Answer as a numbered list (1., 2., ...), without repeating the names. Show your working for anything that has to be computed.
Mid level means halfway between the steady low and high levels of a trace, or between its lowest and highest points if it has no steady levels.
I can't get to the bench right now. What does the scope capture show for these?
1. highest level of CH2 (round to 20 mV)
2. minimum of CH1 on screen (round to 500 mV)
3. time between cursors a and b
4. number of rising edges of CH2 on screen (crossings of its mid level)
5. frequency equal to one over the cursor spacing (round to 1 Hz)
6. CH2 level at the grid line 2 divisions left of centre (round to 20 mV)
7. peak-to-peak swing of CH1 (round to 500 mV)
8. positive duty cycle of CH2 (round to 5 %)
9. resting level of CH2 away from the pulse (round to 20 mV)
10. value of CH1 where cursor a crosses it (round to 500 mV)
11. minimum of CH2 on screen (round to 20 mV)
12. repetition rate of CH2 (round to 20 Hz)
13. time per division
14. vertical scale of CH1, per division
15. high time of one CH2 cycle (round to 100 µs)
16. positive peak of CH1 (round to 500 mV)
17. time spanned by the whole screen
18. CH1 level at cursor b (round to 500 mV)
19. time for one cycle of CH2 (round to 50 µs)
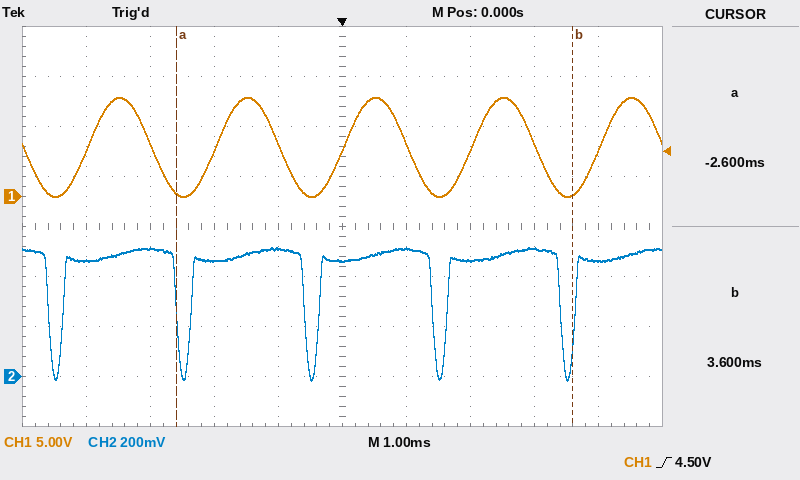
1. 520 mV
2. 0.0 V
3. 3.6 ms − (-2.6 ms) = 6.2 ms
4. 5
5. 1 / 6.2 ms ≈ 161 Hz
6. 460 mV
7. 10.0 V − (0.0 V) = 10.0 V
8. 1.8 ms / 2.00 ms ≈ 90 %
9. 480 mV
10. 500 mV
11. -20 mV
12. 1 / 2.00 ms ≈ 500 Hz
13. 1 ms
14. 5 V
15. 1.8 ms
16. 10.0 V
17. 10 ms
18. 0.0 V
19. 2.00 ms
